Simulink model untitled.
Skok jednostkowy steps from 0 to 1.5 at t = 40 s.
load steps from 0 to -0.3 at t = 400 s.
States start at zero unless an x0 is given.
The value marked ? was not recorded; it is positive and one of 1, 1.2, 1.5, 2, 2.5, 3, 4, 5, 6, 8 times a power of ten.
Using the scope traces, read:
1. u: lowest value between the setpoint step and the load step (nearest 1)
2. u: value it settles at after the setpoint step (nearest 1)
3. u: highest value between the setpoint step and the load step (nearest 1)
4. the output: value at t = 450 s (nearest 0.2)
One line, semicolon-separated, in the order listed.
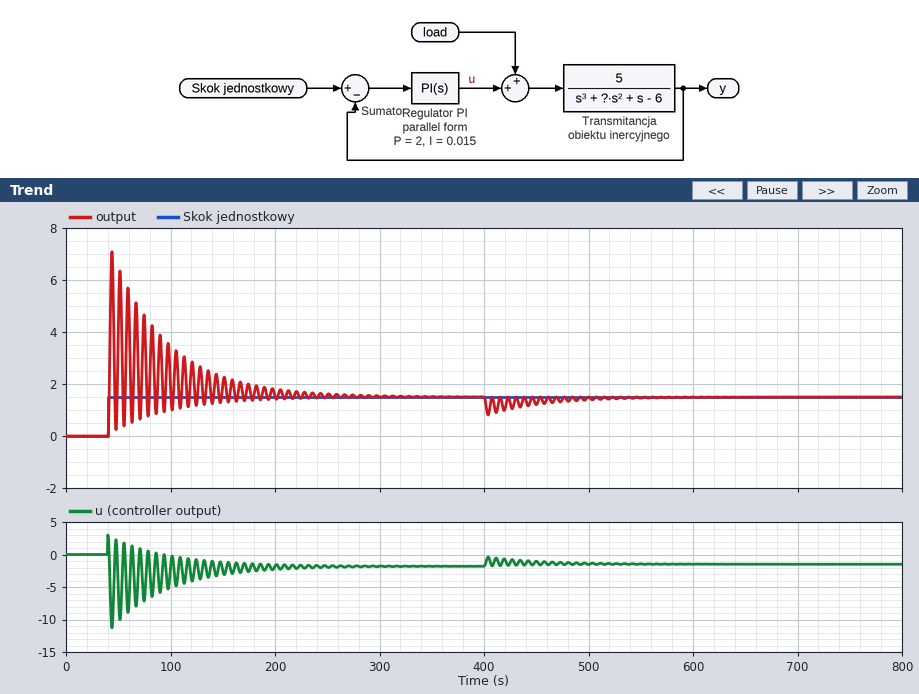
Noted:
-11; -2; 3; 1.2
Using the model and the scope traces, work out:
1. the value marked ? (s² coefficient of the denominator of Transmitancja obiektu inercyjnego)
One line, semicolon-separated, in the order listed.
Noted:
6
